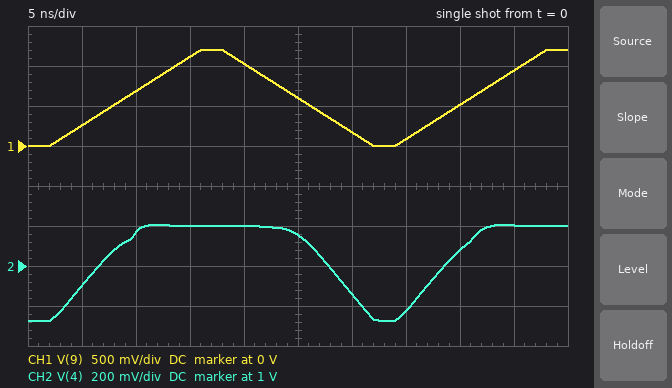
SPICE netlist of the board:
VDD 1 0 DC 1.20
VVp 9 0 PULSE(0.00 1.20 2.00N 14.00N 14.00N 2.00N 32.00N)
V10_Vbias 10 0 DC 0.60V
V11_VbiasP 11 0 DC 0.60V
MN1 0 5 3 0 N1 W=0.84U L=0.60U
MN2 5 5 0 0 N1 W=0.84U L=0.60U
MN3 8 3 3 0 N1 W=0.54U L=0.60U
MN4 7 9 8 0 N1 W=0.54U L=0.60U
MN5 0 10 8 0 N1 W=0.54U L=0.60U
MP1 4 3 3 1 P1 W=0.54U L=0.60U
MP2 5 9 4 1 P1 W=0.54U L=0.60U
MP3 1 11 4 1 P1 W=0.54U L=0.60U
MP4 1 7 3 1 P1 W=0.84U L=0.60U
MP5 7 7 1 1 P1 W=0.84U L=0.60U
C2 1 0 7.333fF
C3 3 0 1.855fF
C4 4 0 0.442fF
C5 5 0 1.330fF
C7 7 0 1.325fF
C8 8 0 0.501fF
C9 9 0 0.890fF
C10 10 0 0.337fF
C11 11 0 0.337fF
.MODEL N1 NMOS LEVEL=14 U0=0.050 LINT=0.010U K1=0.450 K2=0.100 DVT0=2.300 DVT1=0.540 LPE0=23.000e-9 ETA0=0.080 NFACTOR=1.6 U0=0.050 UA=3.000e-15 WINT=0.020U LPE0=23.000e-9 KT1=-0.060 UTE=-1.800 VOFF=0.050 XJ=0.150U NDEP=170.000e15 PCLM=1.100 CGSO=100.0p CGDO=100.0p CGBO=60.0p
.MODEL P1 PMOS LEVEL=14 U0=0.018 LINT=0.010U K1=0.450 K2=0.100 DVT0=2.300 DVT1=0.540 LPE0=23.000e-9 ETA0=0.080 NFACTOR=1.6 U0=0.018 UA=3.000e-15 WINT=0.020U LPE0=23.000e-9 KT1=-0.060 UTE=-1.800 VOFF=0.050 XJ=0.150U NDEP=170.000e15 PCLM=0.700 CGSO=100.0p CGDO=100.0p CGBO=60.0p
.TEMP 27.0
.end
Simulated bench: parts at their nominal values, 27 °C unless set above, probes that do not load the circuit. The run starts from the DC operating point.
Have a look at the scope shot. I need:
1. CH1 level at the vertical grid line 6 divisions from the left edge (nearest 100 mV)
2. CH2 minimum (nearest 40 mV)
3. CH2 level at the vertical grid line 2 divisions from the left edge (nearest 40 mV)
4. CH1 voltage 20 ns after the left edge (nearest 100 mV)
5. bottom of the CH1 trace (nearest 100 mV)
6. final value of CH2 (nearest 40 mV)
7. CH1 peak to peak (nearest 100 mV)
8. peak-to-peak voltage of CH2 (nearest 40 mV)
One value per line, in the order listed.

200 mV
720 mV
1.16 V
1.0 V
0 V
1.20 V
1.2 V
480 mV
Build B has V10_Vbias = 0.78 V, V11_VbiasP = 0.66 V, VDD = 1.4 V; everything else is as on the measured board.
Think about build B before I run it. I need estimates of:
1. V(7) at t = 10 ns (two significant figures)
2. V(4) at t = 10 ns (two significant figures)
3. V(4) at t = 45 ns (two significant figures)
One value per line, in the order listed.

780 mV
1.3 V
1.4 V
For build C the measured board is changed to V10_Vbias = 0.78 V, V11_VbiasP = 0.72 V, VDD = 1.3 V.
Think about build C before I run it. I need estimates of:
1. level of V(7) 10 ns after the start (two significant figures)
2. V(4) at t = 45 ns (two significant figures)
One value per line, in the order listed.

680 mV
1.3 V
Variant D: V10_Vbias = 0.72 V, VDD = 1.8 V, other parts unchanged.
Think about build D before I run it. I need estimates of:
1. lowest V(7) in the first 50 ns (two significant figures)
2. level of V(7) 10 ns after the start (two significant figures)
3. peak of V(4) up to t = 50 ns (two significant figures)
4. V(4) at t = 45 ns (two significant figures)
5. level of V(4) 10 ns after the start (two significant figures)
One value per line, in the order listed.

1.1 V
1.2 V
1.8 V
1.7 V
1.5 V
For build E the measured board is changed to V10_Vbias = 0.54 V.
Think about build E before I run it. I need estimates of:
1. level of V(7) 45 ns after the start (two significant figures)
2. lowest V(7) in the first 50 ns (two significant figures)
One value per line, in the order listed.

660 mV
650 mV
